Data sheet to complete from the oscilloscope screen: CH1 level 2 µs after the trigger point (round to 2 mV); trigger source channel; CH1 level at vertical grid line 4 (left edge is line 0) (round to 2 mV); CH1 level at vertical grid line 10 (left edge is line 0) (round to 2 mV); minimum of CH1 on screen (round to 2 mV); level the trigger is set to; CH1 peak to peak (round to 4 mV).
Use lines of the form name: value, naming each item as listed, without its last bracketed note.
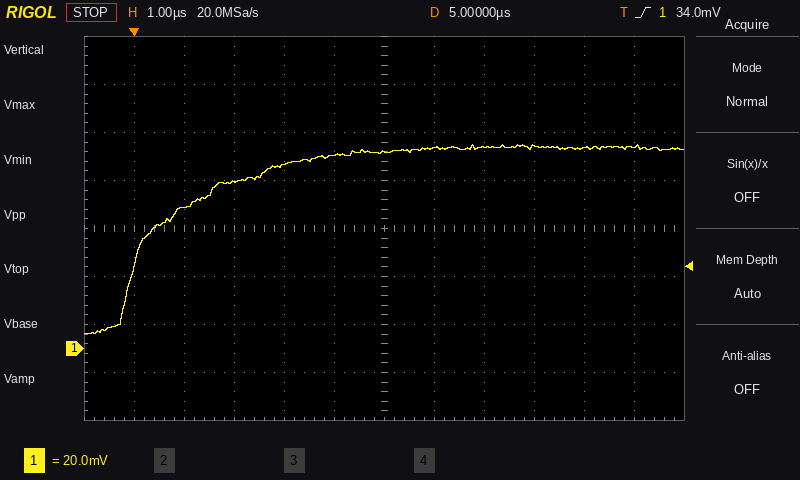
CH1 level 2 µs after the trigger point: 70 mV
trigger source channel: CH1
CH1 level at vertical grid line 4 (left edge is line 0): 76 mV
CH1 level at vertical grid line 10 (left edge is line 0): 84 mV
minimum of CH1 on screen: 6 mV
level the trigger is set to: 34.0 mV
CH1 peak to peak: 80 mV
